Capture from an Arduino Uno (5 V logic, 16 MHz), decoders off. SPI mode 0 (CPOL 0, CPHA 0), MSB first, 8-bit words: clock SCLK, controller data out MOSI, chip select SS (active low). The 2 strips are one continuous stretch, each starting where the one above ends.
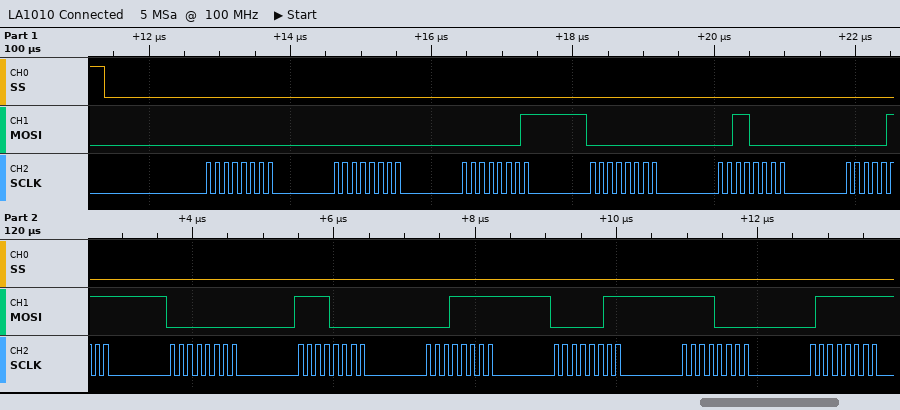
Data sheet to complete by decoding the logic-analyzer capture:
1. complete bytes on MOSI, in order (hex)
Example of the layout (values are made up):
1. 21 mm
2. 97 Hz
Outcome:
1. 00 00 01 00 30 07 00 F0 1F 03 F0 7F
